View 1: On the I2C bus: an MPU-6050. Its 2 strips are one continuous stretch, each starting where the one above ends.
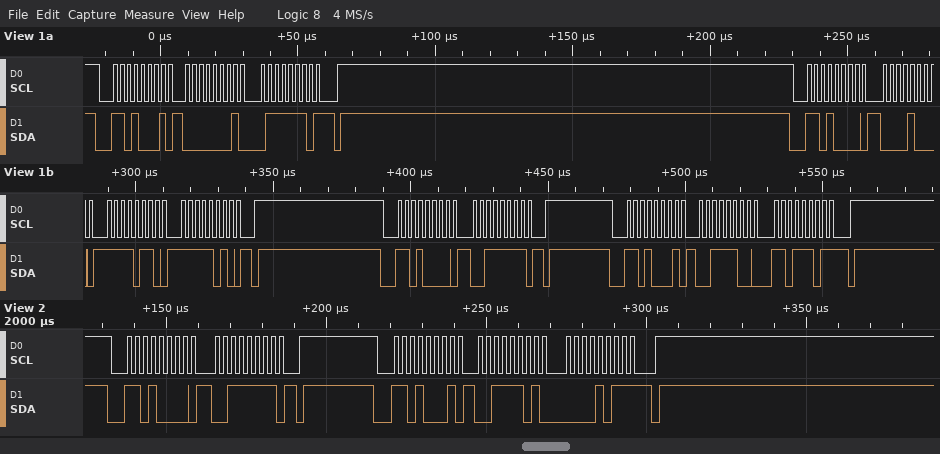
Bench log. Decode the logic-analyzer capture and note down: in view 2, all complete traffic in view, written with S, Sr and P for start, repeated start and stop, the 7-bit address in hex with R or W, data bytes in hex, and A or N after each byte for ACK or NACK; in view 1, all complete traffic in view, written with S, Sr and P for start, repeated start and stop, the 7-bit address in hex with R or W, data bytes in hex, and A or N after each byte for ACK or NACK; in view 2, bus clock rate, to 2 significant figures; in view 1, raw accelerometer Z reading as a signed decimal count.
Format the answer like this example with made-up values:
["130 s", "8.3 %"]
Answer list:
["S 68W A 3F A P S 68R A 3D A 0B N P", "S 68R A 01 A 7E N P S 68W A 08 A F6 A FA A P S 68W A 3F A P S 68R A 3C A DD N P", "400 kHz", "15581"]
